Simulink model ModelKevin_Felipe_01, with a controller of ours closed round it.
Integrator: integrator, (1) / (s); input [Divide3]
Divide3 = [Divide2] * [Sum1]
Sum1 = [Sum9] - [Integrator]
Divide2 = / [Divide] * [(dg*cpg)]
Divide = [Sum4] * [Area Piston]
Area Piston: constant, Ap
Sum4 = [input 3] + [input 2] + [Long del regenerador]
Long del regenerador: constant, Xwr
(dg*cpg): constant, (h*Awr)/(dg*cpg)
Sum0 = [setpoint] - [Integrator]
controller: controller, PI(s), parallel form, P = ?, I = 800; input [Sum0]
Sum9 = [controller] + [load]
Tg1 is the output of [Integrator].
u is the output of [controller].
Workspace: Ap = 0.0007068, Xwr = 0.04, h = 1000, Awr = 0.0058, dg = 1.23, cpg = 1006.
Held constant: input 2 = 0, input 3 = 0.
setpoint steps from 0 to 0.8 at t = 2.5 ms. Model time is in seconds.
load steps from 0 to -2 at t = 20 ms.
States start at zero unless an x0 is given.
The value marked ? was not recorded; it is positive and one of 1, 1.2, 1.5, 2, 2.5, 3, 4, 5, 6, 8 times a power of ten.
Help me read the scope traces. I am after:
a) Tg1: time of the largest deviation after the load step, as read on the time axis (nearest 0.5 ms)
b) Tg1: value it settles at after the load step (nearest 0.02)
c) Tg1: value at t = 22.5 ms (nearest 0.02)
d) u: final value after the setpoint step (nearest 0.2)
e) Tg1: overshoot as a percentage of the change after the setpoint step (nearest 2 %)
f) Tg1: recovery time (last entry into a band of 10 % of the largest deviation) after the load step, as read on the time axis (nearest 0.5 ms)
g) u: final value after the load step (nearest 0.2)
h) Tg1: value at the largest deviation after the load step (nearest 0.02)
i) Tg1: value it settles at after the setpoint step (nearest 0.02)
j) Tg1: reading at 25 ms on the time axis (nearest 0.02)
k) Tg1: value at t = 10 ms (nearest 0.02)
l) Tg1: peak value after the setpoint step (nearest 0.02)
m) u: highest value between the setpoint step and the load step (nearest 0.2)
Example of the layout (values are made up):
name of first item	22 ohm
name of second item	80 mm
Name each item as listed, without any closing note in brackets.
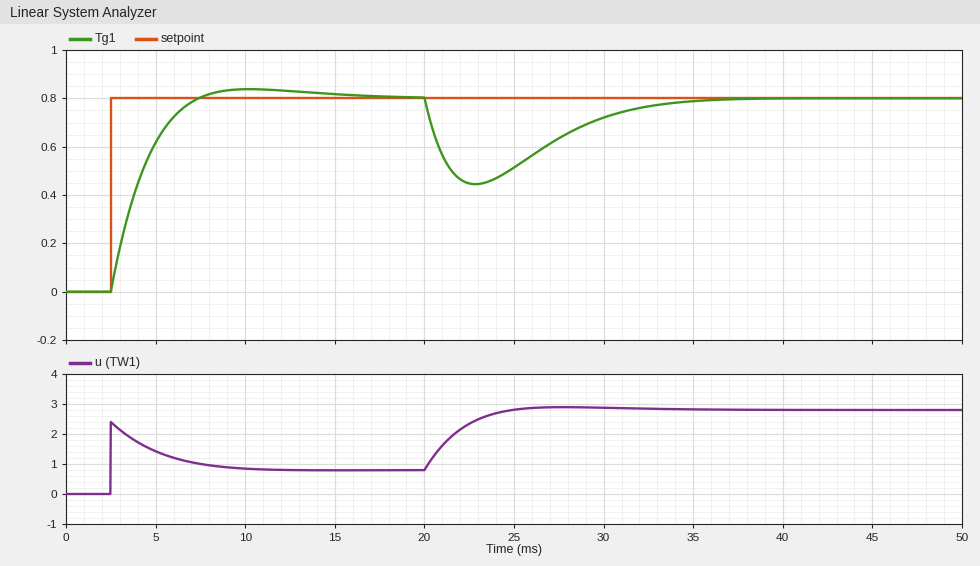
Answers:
Tg1: time of the largest deviation after the load step, as read on the time axis	23.0 ms
Tg1: value it settles at after the load step	0.80
Tg1: value at t = 22.5 ms	0.44
u: final value after the setpoint step	0.8
Tg1: overshoot as a percentage of the change after the setpoint step	4 %
Tg1: recovery time (last entry into a band of 10 % of the largest deviation) after the load step, as read on the time axis	32.5 ms
u: final value after the load step	2.8
Tg1: value at the largest deviation after the load step	0.44
Tg1: value it settles at after the setpoint step	0.80
Tg1: reading at 25 ms on the time axis	0.52
Tg1: value at t = 10 ms	0.84
Tg1: peak value after the setpoint step	0.84
u: highest value between the setpoint step and the load step	2.4
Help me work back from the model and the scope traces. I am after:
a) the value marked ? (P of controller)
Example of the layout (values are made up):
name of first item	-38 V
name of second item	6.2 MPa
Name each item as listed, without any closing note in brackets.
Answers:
the value marked ?	3
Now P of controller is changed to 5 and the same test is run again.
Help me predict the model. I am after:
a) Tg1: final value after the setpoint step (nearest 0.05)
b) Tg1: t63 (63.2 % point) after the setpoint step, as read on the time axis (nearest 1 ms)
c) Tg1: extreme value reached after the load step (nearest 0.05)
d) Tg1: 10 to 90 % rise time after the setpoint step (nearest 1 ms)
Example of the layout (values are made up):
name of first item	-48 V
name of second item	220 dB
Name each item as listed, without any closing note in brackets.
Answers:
Tg1: final value after the setpoint step	0.80
Tg1: t63 (63.2 % point) after the setpoint step, as read on the time axis	4 ms
Tg1: extreme value reached after the load step	0.55
Tg1: 10 to 90 % rise time after the setpoint step	3 ms
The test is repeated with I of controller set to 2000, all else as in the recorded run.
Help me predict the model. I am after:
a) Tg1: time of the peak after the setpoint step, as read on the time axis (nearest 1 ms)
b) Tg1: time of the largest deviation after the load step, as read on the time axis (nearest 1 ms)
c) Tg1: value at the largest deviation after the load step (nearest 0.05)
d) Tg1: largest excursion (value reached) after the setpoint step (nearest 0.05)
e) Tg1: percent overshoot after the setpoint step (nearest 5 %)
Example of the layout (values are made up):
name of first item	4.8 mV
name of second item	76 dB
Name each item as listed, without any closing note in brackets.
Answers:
Tg1: time of the peak after the setpoint step, as read on the time axis	7 ms
Tg1: time of the largest deviation after the load step, as read on the time axis	22 ms
Tg1: value at the largest deviation after the load step	0.50
Tg1: largest excursion (value reached) after the setpoint step	0.95
Tg1: percent overshoot after the setpoint step	20 %
